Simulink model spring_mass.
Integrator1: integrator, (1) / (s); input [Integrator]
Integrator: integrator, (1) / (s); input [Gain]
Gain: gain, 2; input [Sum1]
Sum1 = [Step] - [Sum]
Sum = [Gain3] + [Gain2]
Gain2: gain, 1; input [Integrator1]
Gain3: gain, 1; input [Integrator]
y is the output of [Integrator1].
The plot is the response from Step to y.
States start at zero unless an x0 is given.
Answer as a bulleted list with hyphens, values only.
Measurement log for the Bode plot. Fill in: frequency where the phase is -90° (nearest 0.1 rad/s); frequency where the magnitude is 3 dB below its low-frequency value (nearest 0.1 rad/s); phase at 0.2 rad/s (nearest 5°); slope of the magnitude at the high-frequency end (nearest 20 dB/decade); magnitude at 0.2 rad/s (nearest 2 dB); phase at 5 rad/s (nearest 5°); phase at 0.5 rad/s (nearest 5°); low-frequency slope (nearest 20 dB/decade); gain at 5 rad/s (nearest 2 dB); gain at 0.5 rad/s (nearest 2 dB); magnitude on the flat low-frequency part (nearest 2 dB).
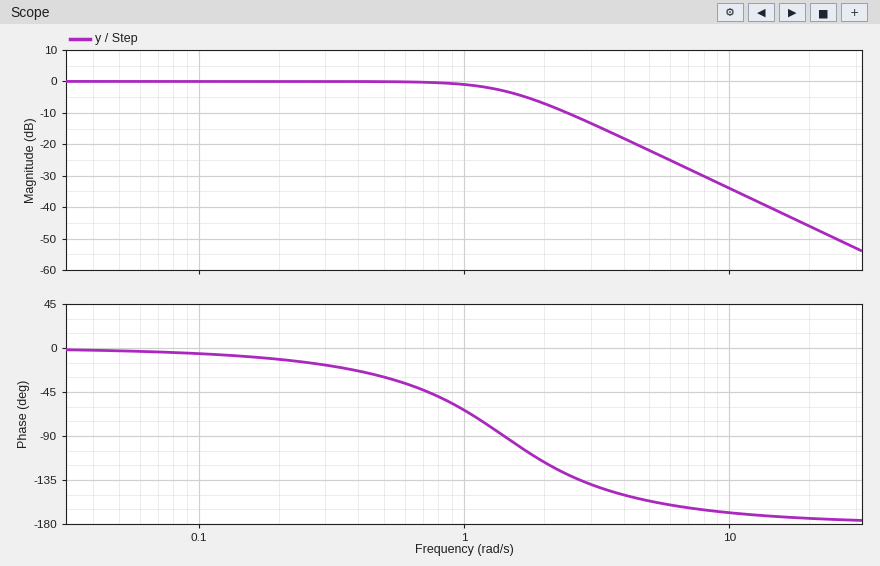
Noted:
- 1.4 rad/s
- 1.4 rad/s
- -10°
- -40 dB/decade
- 0 dB
- -155°
- -30°
- 0 dB/decade
- -22 dB
- 0 dB
- 0 dB
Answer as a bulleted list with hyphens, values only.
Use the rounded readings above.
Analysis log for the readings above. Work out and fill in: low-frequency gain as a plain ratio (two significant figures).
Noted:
- 1.0
